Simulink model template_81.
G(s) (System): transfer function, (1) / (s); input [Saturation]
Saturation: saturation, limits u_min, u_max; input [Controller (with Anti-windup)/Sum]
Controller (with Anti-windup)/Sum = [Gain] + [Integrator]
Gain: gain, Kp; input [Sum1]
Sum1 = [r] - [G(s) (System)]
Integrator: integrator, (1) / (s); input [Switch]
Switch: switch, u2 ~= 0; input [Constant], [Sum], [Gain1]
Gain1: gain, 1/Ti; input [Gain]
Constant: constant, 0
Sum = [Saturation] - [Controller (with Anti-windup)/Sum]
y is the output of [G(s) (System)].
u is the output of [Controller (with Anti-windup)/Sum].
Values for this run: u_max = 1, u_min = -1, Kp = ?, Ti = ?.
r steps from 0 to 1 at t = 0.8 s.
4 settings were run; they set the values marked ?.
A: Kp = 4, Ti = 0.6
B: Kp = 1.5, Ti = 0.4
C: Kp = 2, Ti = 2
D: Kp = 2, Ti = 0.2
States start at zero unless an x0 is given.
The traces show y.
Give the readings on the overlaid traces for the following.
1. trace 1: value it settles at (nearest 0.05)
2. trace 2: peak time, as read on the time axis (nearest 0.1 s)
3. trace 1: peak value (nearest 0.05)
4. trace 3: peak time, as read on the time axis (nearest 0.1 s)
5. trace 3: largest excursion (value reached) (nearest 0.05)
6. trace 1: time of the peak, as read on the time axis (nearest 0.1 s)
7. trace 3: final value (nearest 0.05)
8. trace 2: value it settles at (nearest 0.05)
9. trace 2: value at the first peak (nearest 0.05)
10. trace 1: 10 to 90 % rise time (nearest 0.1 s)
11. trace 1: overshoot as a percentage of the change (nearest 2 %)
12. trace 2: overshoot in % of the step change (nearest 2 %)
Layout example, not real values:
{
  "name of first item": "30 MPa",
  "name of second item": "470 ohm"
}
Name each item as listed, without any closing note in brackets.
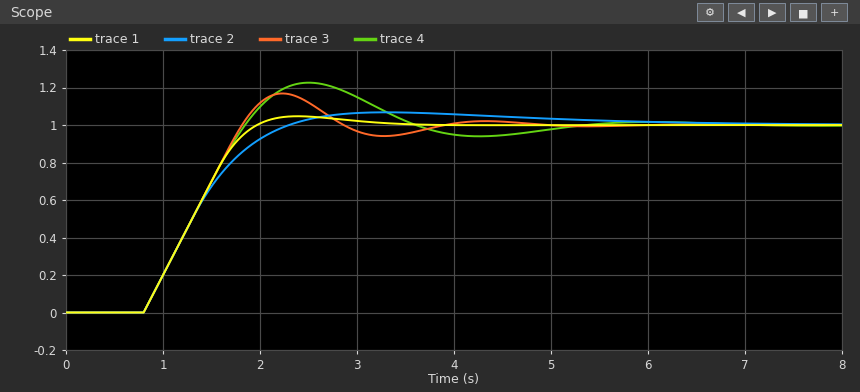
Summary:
{
  "trace 1: value it settles at": "1.00",
  "trace 2: peak time, as read on the time axis": "3.3 s",
  "trace 1: peak value": "1.05",
  "trace 3: peak time, as read on the time axis": "2.2 s",
  "trace 3: largest excursion (value reached)": "1.15",
  "trace 1: time of the peak, as read on the time axis": "2.4 s",
  "trace 3: final value": "1.00",
  "trace 2: value it settles at": "1.00",
  "trace 2: value at the first peak": "1.05",
  "trace 1: 10 to 90 % rise time": "0.8 s",
  "trace 1: overshoot as a percentage of the change": "4 %",
  "trace 2: overshoot in % of the step change": "6 %"
}
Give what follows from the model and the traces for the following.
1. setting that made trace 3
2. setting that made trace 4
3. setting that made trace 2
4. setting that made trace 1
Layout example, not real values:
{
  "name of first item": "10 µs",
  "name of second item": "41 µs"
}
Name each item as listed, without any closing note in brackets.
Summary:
{
  "setting that made trace 3": "D",
  "setting that made trace 4": "B",
  "setting that made trace 2": "C",
  "setting that made trace 1": "A"
}
